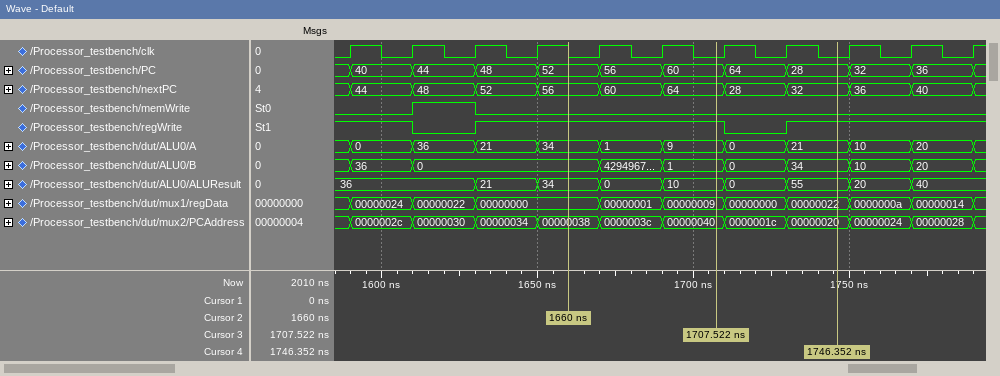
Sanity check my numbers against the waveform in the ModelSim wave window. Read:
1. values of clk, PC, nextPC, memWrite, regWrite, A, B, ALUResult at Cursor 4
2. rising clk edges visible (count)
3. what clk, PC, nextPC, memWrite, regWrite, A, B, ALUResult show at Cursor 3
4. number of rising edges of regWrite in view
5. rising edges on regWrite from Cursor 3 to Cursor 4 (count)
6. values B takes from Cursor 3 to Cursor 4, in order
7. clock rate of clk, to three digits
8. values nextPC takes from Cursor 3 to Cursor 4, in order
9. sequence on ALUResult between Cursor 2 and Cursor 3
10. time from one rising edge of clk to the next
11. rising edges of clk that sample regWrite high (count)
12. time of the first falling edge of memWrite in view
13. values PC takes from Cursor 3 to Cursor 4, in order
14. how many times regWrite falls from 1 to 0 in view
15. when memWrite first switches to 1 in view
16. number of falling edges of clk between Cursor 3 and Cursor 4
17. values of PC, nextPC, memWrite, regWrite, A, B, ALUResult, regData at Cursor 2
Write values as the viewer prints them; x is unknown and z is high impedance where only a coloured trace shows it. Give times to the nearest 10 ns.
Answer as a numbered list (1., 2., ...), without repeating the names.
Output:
1. clk=0, PC=28, nextPC=32, memWrite=0, regWrite=1, A=21, B=34, ALUResult=55
2. 11
3. clk=0, PC=60, nextPC=64, memWrite=0, regWrite=1, A=9, B=1, ALUResult=10
4. 2
5. 1
6. 1, 0, 34
7. 50.0 MHz
8. 64, 28, 32
9. 34, 0, 10
10. 20 ns
11. 9
12. 1630 ns
13. 60, 64, 28
14. 2
15. 1610 ns
16. 2
17. PC=52, nextPC=56, memWrite=0, regWrite=1, A=34, B=0, ALUResult=34, regData=00000000
